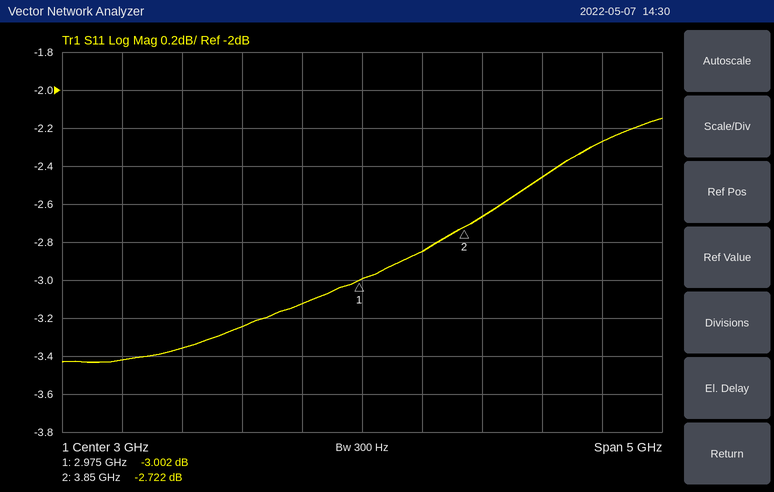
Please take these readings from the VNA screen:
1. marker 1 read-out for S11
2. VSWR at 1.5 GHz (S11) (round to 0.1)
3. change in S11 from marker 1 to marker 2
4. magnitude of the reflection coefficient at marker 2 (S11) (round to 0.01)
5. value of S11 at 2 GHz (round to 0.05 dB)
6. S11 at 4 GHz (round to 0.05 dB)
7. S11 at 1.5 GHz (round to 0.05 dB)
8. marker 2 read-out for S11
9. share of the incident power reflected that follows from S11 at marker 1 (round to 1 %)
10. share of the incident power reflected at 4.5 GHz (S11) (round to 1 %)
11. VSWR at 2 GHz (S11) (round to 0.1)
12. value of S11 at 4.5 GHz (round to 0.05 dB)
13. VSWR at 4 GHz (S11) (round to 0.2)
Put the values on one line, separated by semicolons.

-3.002 dB; 5.2; 0.280 dB; 0.73; -3.25 dB; -2.65 dB; -3.35 dB; -2.722 dB; 50 %; 57 %; 5.4; -2.45 dB; 6.6
